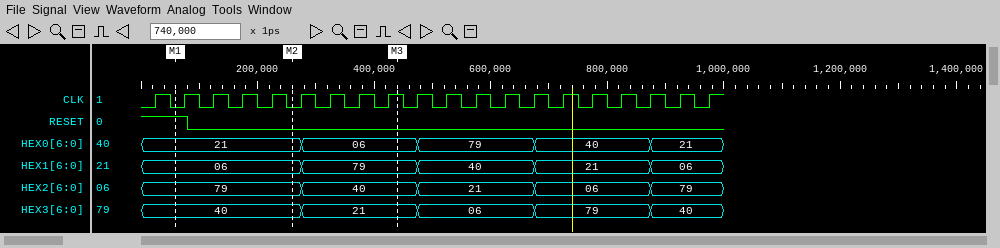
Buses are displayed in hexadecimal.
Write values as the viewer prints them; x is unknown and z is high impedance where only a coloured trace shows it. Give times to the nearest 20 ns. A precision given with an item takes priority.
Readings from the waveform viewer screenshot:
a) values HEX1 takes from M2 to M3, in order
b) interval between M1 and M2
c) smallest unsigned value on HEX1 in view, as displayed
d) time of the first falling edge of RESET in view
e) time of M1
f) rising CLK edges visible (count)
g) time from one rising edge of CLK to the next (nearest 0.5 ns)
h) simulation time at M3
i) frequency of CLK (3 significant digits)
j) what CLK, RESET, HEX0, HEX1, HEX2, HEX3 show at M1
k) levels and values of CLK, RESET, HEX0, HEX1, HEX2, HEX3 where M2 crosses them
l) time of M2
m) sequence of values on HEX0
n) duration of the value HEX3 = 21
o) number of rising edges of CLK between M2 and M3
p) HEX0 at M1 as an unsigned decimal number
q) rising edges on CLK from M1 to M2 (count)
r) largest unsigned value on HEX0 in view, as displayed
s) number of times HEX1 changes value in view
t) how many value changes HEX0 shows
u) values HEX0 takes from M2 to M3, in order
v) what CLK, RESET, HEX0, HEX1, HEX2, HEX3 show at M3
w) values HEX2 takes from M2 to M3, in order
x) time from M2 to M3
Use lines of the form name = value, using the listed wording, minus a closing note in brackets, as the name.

values HEX1 takes from M2 to M3, in order = 06, 79
interval between M1 and M2 = 200 ns
smallest unsigned value on HEX1 in view, as displayed = 06
time of the first falling edge of RESET in view = 80 ns
time of M1 = 60 ns
rising CLK edges visible = 20
time from one rising edge of CLK to the next = 50 ns
simulation time at M3 = 440 ns
frequency of CLK = 20.0 MHz
what CLK, RESET, HEX0, HEX1, HEX2, HEX3 show at M1 = CLK=0, RESET=1, HEX0=21, HEX1=06, HEX2=79, HEX3=40
levels and values of CLK, RESET, HEX0, HEX1, HEX2, HEX3 where M2 crosses them = CLK=0, RESET=0, HEX0=21, HEX1=06, HEX2=79, HEX3=40
time of M2 = 260 ns
sequence of values on HEX0 = 21, 06, 79, 40, 21
duration of the value HEX3 = 21 = 200 ns
number of rising edges of CLK between M2 and M3 = 4
HEX0 at M1 as an unsigned decimal number = 33
rising edges on CLK from M1 to M2 = 4
largest unsigned value on HEX0 in view, as displayed = 79
number of times HEX1 changes value in view = 4
how many value changes HEX0 shows = 4
values HEX0 takes from M2 to M3, in order = 21, 06
what CLK, RESET, HEX0, HEX1, HEX2, HEX3 show at M3 = CLK=1, RESET=0, HEX0=06, HEX1=79, HEX2=40, HEX3=21
values HEX2 takes from M2 to M3, in order = 79, 40
time from M2 to M3 = 180 ns
